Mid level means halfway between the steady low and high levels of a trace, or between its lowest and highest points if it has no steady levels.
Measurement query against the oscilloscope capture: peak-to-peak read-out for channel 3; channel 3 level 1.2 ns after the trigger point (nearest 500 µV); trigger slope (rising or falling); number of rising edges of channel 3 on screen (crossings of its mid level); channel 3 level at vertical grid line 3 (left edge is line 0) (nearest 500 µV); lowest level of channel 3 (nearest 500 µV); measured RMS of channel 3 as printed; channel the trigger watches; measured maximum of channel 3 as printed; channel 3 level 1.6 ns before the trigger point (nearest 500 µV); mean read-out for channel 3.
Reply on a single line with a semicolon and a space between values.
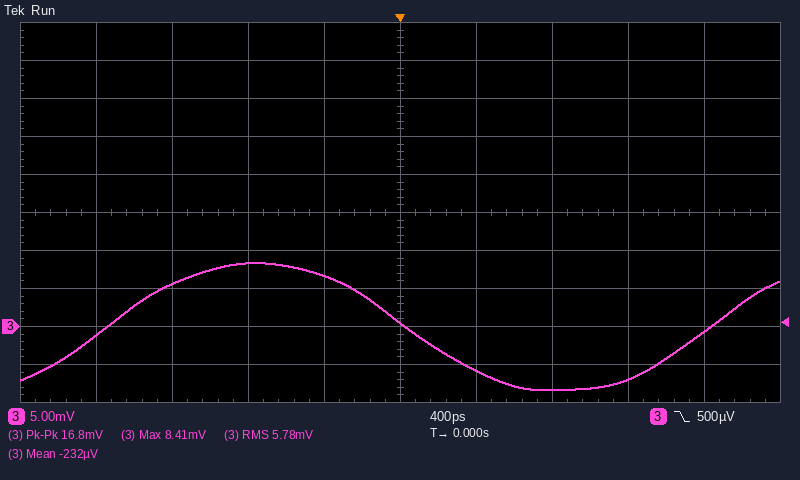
16.8 mV; -7.0 mV; falling; 2; 8.5 mV; -8.5 mV; 5.78 mV; channel 3; 8.41 mV; -1.0 mV; -232 µV
